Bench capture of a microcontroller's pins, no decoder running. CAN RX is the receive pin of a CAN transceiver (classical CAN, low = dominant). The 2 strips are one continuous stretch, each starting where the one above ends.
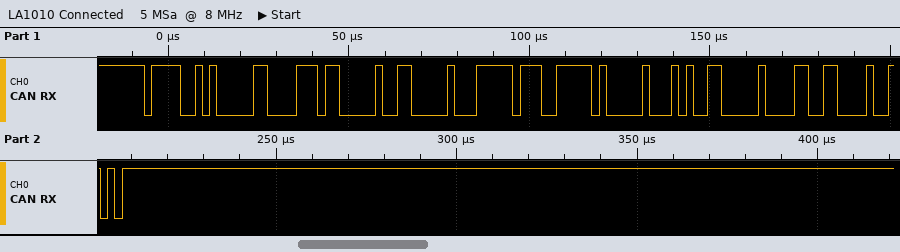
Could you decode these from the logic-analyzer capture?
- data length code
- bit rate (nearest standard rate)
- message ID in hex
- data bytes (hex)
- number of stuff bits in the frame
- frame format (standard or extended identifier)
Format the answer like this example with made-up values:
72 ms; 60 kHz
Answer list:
8; 500 kbit/s; 0x794; 76 03 00 FF 3F 00 A6 00; 7; standard
